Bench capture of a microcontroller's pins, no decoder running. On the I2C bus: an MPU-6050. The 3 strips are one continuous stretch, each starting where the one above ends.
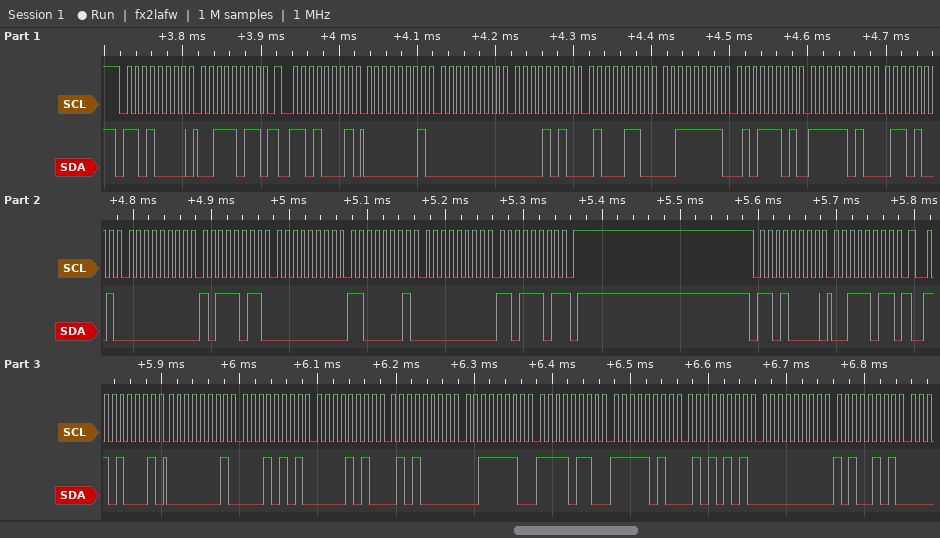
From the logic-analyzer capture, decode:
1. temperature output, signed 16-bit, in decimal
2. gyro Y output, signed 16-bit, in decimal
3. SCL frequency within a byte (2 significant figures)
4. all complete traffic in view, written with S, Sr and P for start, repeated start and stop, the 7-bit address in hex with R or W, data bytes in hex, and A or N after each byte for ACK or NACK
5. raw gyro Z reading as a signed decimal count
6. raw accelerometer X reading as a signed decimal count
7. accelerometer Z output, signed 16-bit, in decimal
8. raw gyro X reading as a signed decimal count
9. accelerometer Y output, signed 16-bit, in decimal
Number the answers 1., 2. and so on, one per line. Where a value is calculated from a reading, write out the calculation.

1. 0xFA69 = -1431
2. 0x00C1 = 193
3. 100 kHz
4. S 68W A 3B A Sr 68R A 01 A 00 A 0A A 46 A 3F A 5D A FA A 69 A 00 A BB A 00 A C1 A 00 A DD N P S 68W A 3B A Sr 68R A 01 A 15 A 0A A 50 A 3E A F6 A FA A 55 A 00 A A5 A
5. 0x00DD = 221
6. 0x0100 = 256
7. 0x3F5D = 16221
8. 0x00BB = 187
9. 0x0A46 = 2630
